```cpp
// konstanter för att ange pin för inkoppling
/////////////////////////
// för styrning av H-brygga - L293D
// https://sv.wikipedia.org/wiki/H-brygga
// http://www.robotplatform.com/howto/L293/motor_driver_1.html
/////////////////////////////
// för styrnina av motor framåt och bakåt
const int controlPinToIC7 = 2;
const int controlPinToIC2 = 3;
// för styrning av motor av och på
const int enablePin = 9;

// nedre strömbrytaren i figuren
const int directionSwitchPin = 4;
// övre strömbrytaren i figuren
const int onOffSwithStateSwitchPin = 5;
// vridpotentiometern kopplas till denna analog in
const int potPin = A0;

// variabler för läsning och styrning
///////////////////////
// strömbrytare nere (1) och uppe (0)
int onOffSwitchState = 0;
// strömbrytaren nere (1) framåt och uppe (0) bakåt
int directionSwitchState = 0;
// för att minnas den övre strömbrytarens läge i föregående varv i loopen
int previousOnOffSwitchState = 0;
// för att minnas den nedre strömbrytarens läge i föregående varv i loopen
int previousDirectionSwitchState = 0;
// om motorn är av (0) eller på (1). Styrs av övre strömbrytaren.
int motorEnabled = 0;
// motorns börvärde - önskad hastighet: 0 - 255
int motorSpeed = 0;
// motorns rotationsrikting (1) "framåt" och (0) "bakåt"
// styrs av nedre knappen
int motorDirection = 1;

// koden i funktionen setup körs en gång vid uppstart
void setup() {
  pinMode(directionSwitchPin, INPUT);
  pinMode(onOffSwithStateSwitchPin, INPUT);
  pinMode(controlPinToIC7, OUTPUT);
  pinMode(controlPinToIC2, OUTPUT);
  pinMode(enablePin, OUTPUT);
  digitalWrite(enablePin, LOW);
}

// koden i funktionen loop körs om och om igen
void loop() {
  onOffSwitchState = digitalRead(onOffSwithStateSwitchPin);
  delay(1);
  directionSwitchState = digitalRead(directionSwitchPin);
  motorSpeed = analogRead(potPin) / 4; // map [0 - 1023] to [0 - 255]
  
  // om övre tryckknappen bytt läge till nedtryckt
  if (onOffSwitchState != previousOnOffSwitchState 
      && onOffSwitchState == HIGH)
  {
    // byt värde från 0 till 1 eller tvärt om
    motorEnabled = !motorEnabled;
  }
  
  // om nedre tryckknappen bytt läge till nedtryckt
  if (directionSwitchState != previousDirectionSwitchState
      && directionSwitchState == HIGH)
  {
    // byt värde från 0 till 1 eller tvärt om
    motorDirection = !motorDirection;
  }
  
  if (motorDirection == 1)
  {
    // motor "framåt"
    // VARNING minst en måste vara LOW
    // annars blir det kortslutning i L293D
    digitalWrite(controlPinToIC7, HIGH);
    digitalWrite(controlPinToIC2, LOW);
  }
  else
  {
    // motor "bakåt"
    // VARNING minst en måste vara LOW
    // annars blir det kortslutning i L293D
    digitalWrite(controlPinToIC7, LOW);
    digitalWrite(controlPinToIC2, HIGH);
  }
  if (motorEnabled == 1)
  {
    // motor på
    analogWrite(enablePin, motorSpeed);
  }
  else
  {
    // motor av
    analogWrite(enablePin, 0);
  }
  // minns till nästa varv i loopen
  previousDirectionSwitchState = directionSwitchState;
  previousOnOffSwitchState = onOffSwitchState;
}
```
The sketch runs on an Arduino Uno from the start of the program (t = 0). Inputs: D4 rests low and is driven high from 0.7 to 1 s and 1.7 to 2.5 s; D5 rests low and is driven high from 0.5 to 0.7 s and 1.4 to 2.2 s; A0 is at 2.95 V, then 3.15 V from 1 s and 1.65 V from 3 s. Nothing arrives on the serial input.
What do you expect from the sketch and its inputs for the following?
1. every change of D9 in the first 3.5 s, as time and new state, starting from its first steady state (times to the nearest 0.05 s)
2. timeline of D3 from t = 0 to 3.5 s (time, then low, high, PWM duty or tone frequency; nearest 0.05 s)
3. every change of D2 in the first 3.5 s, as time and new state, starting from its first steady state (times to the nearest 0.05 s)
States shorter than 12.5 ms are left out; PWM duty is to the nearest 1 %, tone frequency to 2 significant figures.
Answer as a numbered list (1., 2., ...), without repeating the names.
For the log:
1. 0 s low; 0.5 s PWM 59 %; 1 s PWM 63 %; 1.4 s low
2. 0 s low; 0.7 s high; 1.7 s low
3. 0 s high; 0.7 s low; 1.7 s high
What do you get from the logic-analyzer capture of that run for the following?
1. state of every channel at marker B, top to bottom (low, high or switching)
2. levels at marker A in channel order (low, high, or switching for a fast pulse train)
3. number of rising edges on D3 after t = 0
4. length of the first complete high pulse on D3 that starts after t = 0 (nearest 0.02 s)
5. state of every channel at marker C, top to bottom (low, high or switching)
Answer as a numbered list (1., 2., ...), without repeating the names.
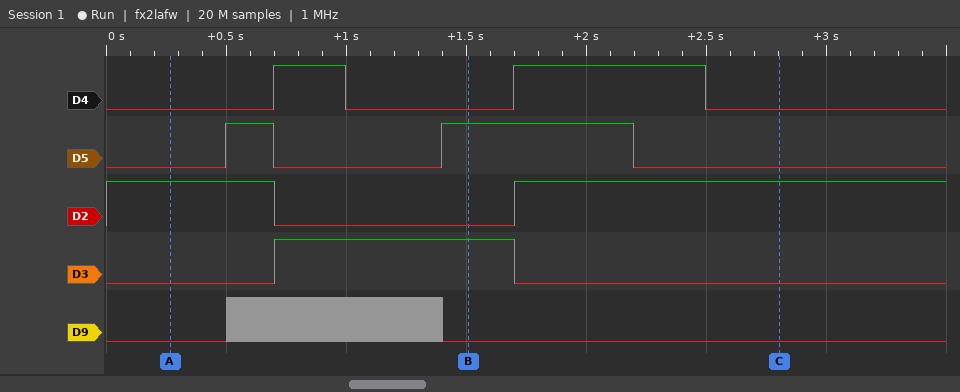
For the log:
1. D4 low, D5 high, D2 low, D3 high, D9 low
2. D4 low, D5 low, D2 high, D3 low, D9 low
3. 1
4. 1.00 s
5. D4 low, D5 low, D2 high, D3 low, D9 low
